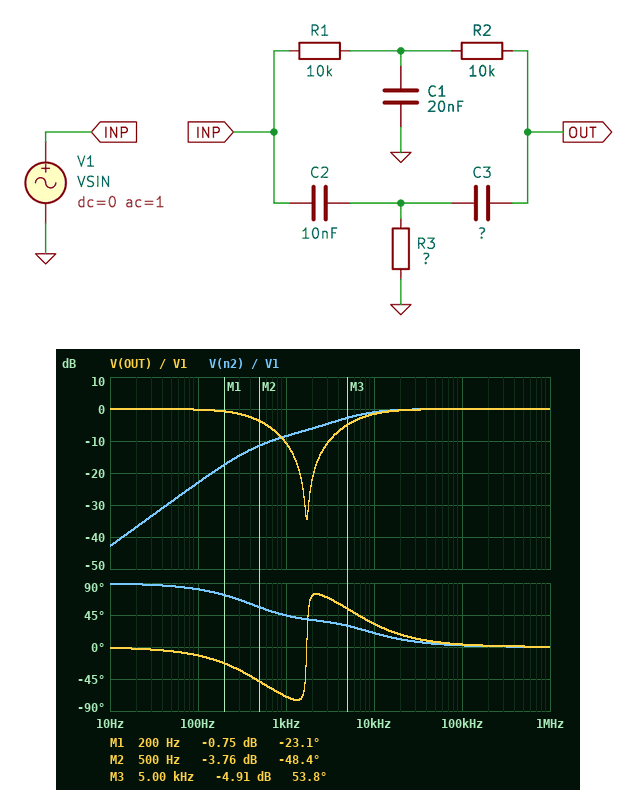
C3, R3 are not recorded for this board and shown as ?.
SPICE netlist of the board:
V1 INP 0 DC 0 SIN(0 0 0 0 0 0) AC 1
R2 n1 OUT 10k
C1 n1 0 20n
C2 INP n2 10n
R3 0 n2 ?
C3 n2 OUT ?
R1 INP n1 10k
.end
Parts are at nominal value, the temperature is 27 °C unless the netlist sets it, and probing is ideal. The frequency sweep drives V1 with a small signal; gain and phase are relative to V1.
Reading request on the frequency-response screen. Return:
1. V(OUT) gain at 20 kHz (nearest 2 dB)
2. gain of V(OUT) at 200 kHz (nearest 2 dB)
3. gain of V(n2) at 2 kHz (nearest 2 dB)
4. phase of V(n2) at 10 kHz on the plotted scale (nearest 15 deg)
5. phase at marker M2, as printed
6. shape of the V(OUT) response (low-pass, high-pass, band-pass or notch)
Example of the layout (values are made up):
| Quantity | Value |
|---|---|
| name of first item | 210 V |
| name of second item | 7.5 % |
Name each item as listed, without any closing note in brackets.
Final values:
| Quantity | Value |
|---|---|
| V(OUT) gain at 20 kHz | 0 dB |
| gain of V(OUT) at 200 kHz | 0 dB |
| gain of V(n2) at 2 kHz | -6 dB |
| phase of V(n2) at 10 kHz on the plotted scale | 15 deg |
| phase at marker M2, as printed | -48.4 deg |
| shape of the V(OUT) response | notch |
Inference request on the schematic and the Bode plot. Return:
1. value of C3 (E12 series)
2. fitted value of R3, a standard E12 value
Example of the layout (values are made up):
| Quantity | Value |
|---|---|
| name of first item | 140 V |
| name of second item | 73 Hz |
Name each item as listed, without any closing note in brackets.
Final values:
| Quantity | Value |
|---|---|
| value of C3 | 6.8 nF |
| fitted value of R3, a standard E12 value | 6.8 kΩ |
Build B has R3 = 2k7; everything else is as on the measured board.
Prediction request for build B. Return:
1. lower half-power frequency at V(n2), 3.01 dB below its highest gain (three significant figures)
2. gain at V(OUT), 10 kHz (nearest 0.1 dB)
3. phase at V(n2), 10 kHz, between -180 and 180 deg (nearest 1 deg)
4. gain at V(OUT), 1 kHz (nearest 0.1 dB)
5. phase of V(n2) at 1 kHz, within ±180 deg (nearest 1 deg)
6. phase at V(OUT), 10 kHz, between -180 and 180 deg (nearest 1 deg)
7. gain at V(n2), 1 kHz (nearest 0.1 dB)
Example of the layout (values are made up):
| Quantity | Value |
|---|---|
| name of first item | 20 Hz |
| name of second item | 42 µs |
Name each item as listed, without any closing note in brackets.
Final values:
| Quantity | Value |
|---|---|
| lower half-power frequency at V(n2), 3.01 dB below its highest gain | 8.11 kHz |
| gain at V(OUT), 10 kHz | -2.8 dB |
| phase at V(n2), 10 kHz, between -180 and 180 deg | 35 deg |
| gain at V(OUT), 1 kHz | -8.4 dB |
| phase of V(n2) at 1 kHz, within ±180 deg | 61 deg |
| phase at V(OUT), 10 kHz, between -180 and 180 deg | 48 deg |
| gain at V(n2), 1 kHz | -15.1 dB |
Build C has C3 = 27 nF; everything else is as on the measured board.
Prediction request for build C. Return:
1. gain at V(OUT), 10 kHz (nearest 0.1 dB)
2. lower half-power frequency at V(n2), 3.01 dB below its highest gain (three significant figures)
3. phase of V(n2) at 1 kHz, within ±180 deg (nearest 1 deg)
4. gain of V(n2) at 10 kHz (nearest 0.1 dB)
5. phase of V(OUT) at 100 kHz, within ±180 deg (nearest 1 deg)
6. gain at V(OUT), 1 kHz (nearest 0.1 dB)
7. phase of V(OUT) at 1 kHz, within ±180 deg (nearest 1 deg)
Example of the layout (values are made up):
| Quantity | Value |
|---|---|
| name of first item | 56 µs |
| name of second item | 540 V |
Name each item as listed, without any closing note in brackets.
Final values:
| Quantity | Value |
|---|---|
| gain at V(OUT), 10 kHz | -1.0 dB |
| lower half-power frequency at V(n2), 3.01 dB below its highest gain | 4.73 kHz |
| phase of V(n2) at 1 kHz, within ±180 deg | 31 deg |
| gain of V(n2) at 10 kHz | -0.9 dB |
| phase of V(OUT) at 100 kHz, within ±180 deg | 3 deg |
| gain at V(OUT), 1 kHz | -18.8 dB |
| phase of V(OUT) at 1 kHz, within ±180 deg | -7 deg |
